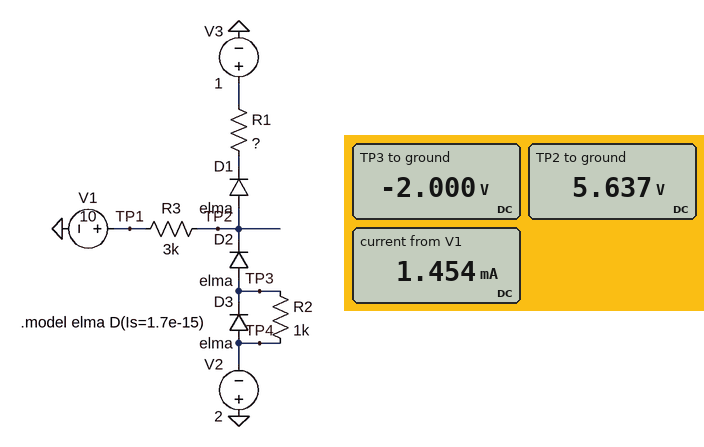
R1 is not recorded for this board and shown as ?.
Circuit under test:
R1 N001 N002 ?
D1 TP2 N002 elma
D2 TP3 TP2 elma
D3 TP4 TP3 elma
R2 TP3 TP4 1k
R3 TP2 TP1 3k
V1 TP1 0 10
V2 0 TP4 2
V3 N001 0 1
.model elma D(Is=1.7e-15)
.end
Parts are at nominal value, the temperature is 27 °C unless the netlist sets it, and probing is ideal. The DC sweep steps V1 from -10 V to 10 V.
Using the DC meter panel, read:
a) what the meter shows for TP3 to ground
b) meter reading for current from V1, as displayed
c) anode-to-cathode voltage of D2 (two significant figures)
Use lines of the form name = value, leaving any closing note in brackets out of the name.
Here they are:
what the meter shows for TP3 to ground = -2.000 V
meter reading for current from V1, as displayed = 1.454 mA
anode-to-cathode voltage of D2 = -7.6 V
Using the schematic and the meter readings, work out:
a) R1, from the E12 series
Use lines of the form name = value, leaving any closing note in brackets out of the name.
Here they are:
R1, from the E12 series = 2.7 kΩ
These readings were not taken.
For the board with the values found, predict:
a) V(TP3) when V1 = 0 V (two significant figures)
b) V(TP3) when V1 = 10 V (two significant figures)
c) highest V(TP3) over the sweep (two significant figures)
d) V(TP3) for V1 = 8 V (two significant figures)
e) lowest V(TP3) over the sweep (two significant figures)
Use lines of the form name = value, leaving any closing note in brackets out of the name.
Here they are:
V(TP3) when V1 = 0 V = -2.0 V
V(TP3) when V1 = 10 V = -2.0 V
highest V(TP3) over the sweep = -2.0 V
V(TP3) for V1 = 8 V = -2.0 V
lowest V(TP3) over the sweep = -2.7 V
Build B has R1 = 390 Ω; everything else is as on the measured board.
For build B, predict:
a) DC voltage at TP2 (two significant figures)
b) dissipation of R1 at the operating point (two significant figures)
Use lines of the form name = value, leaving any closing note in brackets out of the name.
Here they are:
DC voltage at TP2 = 2.7 V
dissipation of R1 at the operating point = 2.3 mW
